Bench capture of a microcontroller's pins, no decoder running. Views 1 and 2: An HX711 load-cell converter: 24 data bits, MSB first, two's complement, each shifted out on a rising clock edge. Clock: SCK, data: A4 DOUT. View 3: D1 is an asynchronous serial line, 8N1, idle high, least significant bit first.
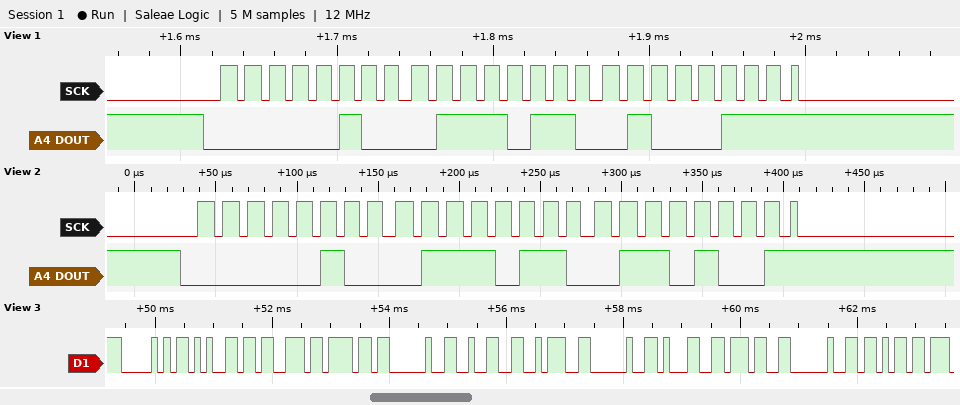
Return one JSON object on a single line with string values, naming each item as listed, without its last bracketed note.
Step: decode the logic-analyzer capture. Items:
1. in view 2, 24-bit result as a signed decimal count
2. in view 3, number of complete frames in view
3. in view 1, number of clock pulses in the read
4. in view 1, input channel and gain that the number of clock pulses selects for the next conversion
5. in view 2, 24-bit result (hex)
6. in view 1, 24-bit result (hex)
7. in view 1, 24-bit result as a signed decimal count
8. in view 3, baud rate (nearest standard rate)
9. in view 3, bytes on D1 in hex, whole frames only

{"in view 2, 24-bit result as a signed decimal count": "292457", "in view 3, number of complete frames in view": "12", "in view 1, number of clock pulses in the read": "25", "in view 1, input channel and gain that the number of clock pulses selects for the next conversion": "channel A, gain 128", "in view 2, 24-bit result": "0x047669", "in view 1, 24-bit result": "0x047647", "in view 1, 24-bit result as a signed decimal count": "292423", "in view 3, baud rate": "9600 baud", "in view 3, bytes on D1 in hex, whole frames only": "0x50 0x65 0x73 0x6F 0x20 0x32 0x3A 0x20 0x31 0x37 0x20 0x6B"}
